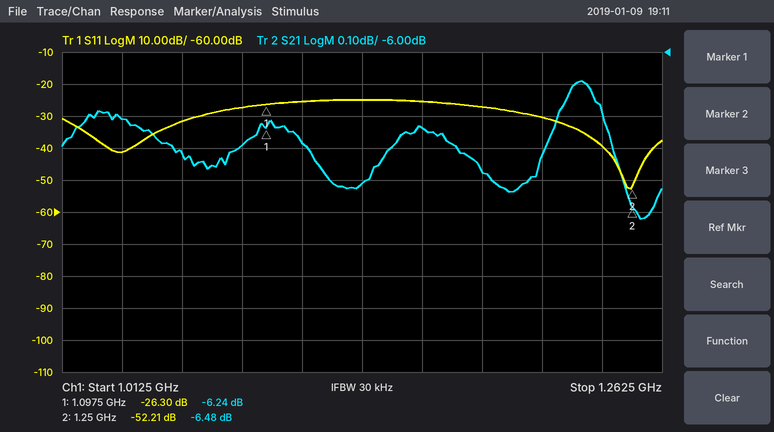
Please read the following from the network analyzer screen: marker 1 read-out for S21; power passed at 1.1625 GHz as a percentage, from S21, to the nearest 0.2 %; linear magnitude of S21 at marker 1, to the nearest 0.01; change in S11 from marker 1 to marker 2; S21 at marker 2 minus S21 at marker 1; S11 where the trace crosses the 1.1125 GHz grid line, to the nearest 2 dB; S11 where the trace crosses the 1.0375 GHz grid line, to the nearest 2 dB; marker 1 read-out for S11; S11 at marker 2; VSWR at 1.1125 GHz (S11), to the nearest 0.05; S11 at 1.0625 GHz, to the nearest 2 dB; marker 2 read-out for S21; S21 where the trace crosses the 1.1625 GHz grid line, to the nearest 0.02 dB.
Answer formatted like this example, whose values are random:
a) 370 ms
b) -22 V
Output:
a) -6.24 dB
b) 23.8 %
c) 0.49
d) -25.91 dB
e) -0.24 dB
f) -26 dB
g) -42 dB
h) -26.30 dB
i) -52.21 dB
j) 1.10
k) -32 dB
l) -6.48 dB
m) -6.24 dB
